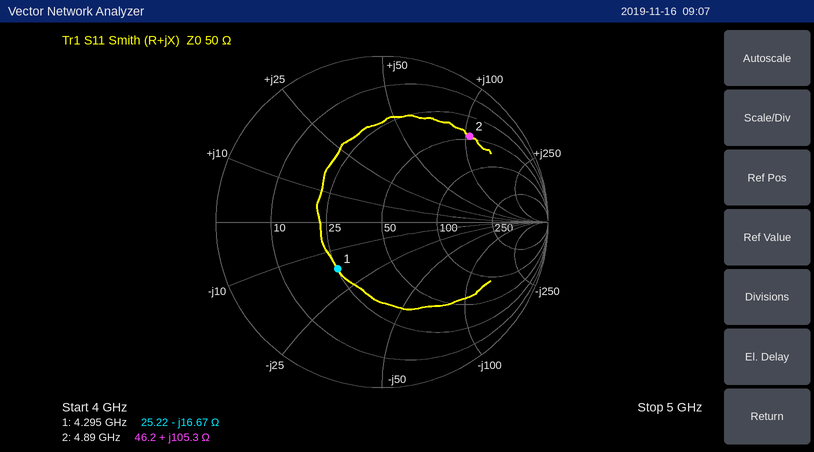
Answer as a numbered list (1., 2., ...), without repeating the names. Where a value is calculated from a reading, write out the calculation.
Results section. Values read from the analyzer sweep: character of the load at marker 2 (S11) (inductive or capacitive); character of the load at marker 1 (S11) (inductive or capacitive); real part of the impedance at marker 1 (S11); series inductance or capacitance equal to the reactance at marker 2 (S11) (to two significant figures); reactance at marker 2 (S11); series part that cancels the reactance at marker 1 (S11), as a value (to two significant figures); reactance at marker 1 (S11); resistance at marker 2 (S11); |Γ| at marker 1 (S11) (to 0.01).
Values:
1. inductive
2. capacitive
3. 25.22 Ω
4. L = 105.3 Ω/(2π × 4.89 GHz) ≈ 3.4 nH
5. +105.3 Ω
6. L = 16.67 Ω/(2π × 4.295 GHz) ≈ 618 pH, so 620 pH to two significant figures
7. -16.67 Ω
8. 46.2 Ω
9. 0.39
